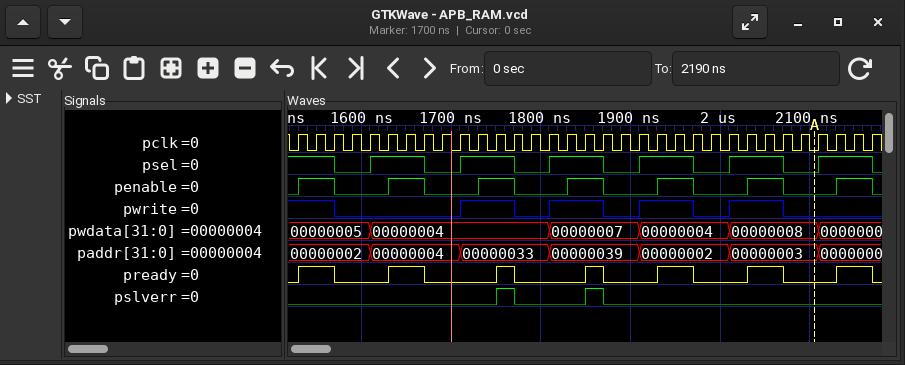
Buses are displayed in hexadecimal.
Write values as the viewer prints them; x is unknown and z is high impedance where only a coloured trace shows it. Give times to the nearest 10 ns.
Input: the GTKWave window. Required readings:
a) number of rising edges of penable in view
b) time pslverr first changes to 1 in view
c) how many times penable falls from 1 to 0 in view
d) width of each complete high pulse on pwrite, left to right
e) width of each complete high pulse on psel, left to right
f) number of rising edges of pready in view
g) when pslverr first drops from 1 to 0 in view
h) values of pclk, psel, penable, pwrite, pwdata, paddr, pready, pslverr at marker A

7
1750 ns
7
60 ns, 60 ns, 60 ns, 60 ns
60 ns, 60 ns, 60 ns, 60 ns, 60 ns, 60 ns
7
1770 ns
pclk=0, psel=0, penable=0, pwrite=0, pwdata=00000008, paddr=00000003, pready=0, pslverr=0
